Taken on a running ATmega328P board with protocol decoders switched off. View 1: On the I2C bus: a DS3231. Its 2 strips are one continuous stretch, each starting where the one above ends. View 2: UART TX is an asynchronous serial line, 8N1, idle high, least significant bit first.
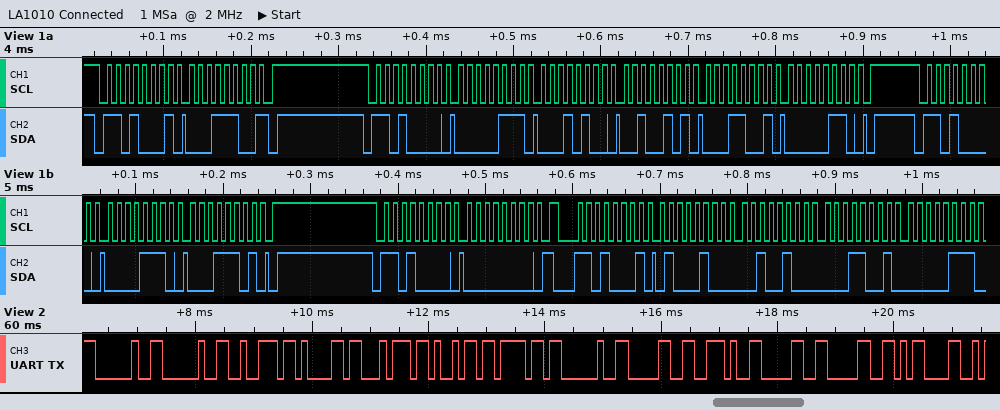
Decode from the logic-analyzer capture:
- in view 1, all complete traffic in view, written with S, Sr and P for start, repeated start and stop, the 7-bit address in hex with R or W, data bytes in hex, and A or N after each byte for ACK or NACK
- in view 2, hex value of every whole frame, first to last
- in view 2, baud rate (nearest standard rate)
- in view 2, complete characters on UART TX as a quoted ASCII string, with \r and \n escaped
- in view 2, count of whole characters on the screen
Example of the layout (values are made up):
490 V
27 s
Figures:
S 68R A 1C N P S 68W A 07 A 14 A 25 A 19 A 06 A P S 68W A 0E A 1D A P S 68W A 00 A Sr 68R A 44 A 24 A 19 A 07 A
20 20 72 61 74 69 6F 20 30 2E 30 30 0D
9600 baud
"  ratio 0.00\r"
13
